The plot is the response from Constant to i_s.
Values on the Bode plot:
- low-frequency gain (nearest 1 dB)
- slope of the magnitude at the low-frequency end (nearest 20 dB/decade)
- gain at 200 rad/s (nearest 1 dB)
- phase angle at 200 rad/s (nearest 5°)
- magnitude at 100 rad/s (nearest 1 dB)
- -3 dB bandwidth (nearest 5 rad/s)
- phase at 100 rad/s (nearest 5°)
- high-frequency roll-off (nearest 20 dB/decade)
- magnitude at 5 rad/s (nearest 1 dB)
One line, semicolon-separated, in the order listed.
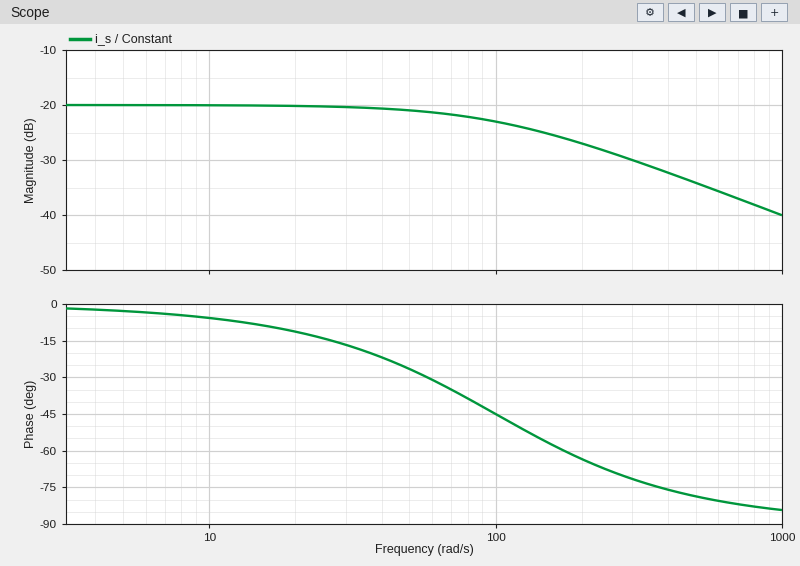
-20 dB; 0 dB/decade; -27 dB; -65°; -23 dB; 100 rad/s; -45°; -20 dB/decade; -20 dB
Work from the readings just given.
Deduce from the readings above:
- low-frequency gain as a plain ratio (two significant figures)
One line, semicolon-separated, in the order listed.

0.10
